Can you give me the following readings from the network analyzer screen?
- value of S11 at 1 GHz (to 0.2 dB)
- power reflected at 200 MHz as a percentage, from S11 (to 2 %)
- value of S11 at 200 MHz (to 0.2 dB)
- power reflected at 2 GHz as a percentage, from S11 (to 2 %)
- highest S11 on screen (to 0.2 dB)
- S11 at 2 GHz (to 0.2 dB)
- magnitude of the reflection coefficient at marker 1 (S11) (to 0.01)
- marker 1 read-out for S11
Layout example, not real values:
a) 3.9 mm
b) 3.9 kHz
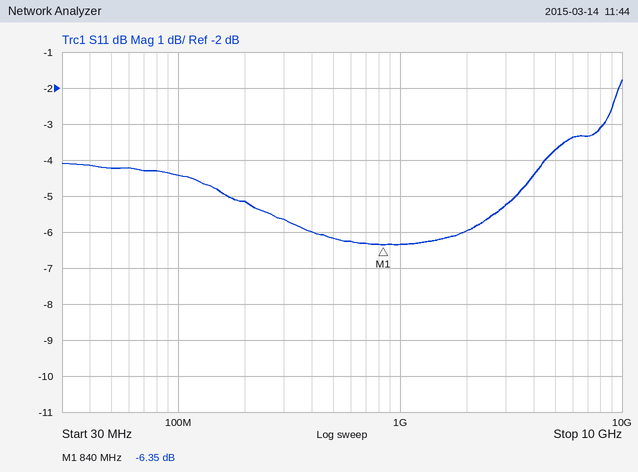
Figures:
a) -6.4 dB
b) 30 %
c) -5.2 dB
d) 26 %
e) -1.8 dB
f) -6.0 dB
g) 0.48
h) -6.35 dB
